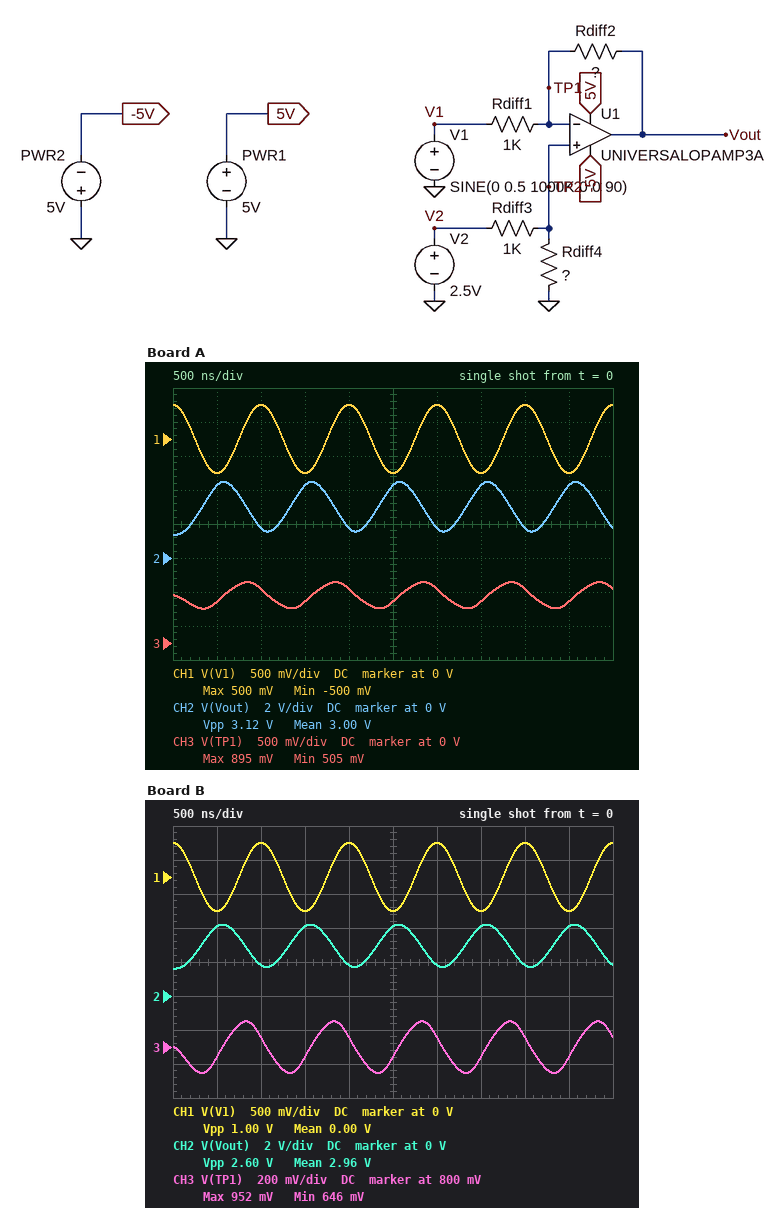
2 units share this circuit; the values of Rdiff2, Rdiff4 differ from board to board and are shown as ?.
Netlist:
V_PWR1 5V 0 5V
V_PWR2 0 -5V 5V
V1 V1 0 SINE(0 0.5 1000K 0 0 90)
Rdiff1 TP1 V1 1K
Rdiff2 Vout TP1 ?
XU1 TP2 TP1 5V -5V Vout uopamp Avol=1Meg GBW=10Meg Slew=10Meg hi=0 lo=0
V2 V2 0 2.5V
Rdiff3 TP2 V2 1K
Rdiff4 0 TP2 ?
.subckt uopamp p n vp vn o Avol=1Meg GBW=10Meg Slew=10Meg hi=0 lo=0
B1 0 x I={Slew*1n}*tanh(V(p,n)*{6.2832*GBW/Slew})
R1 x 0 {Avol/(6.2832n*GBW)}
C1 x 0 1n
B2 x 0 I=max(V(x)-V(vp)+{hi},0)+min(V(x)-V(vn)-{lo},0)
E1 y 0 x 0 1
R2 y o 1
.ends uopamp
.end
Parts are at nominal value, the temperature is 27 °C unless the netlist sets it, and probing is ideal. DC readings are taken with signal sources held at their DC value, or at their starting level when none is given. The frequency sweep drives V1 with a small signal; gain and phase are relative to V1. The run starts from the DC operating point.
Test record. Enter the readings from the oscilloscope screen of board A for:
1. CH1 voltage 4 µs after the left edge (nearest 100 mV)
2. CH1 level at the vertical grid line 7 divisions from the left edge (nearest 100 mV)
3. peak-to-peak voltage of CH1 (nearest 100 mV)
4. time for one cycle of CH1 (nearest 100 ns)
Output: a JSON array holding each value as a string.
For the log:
["500 mV", "-500 mV", "1.0 V", "1.0 µs"]
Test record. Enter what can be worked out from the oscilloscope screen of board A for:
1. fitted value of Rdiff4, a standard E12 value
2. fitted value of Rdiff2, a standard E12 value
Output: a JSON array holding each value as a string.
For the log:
["390 Ω", "3.3 kΩ"]
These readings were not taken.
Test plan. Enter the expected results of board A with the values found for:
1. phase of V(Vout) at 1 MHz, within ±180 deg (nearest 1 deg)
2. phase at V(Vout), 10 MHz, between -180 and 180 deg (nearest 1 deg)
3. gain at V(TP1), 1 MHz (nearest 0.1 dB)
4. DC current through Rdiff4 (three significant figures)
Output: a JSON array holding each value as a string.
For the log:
["157 deg", "103 deg", "-10.4 dB", "1.80 mA"]
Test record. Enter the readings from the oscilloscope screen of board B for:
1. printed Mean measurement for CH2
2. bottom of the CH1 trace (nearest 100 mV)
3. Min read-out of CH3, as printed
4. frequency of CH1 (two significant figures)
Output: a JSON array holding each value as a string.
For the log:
["2.96 V", "-500 mV", "646 mV", "1.0 MHz"]
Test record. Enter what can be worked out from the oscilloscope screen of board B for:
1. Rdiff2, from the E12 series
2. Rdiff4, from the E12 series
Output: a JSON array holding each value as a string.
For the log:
["2.7 kΩ", "470 Ω"]
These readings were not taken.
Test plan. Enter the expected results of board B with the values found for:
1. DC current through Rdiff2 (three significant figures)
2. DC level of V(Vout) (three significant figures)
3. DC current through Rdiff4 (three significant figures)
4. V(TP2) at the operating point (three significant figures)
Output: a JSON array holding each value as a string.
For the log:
["299 µA", "1.61 V", "1.70 mA", "799 mV"]
